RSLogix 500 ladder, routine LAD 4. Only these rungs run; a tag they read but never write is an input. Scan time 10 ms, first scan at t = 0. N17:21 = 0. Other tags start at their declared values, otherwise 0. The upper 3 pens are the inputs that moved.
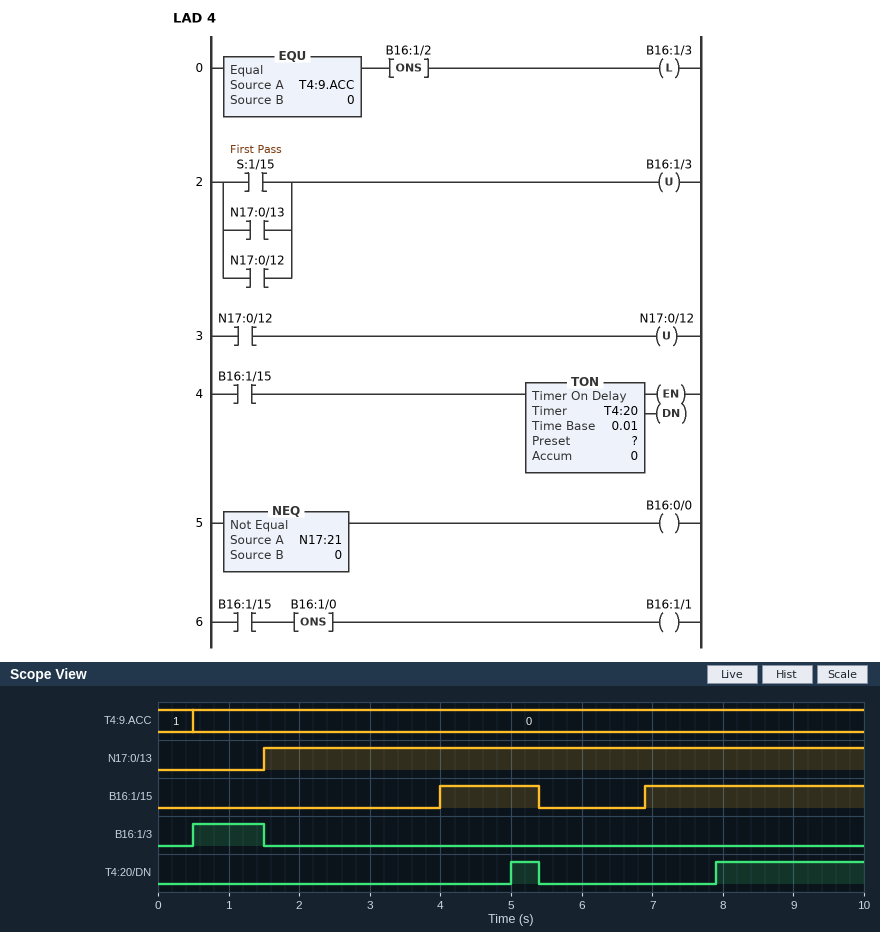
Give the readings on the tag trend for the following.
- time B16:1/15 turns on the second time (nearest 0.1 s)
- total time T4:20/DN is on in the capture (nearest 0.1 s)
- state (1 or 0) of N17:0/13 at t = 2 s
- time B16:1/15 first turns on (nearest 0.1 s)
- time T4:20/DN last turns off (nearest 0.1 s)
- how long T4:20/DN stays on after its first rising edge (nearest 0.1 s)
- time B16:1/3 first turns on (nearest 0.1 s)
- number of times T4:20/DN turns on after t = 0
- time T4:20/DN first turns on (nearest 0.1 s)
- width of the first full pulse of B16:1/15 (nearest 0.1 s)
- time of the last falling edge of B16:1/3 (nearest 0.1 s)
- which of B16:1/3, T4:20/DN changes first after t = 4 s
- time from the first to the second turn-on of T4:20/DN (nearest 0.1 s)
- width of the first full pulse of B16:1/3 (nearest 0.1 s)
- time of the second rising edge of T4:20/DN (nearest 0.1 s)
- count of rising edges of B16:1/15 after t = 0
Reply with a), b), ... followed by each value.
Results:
a) 6.9 s
b) 2.5 s
c) 1
d) 4.0 s
e) 5.4 s
f) 0.4 s
g) 0.5 s
h) 2
i) 5.0 s
j) 1.4 s
k) 1.5 s
l) T4:20/DN
m) 2.9 s
n) 1.0 s
o) 7.9 s
p) 2
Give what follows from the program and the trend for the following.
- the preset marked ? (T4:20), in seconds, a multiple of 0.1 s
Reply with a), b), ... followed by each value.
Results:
a) 1.0 s
